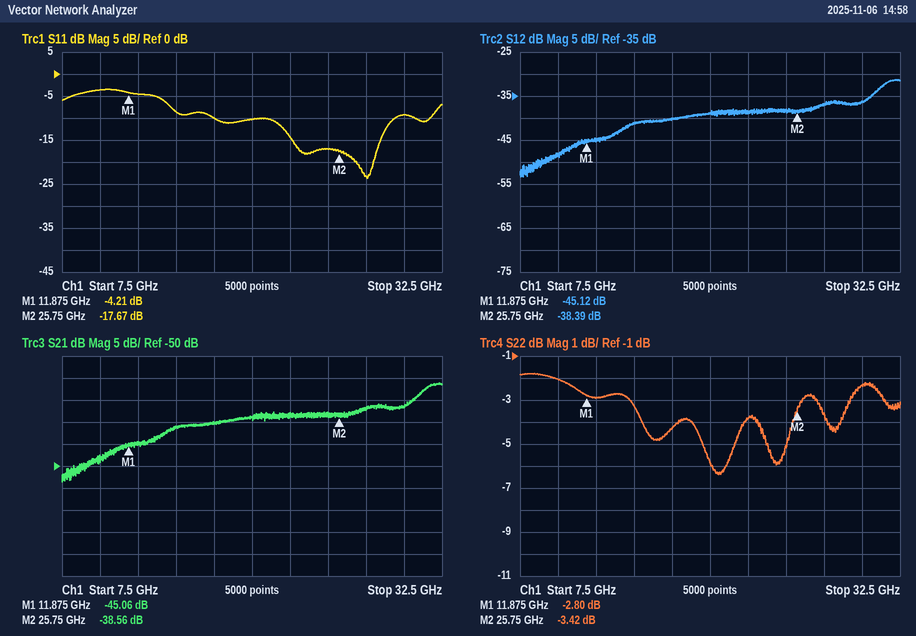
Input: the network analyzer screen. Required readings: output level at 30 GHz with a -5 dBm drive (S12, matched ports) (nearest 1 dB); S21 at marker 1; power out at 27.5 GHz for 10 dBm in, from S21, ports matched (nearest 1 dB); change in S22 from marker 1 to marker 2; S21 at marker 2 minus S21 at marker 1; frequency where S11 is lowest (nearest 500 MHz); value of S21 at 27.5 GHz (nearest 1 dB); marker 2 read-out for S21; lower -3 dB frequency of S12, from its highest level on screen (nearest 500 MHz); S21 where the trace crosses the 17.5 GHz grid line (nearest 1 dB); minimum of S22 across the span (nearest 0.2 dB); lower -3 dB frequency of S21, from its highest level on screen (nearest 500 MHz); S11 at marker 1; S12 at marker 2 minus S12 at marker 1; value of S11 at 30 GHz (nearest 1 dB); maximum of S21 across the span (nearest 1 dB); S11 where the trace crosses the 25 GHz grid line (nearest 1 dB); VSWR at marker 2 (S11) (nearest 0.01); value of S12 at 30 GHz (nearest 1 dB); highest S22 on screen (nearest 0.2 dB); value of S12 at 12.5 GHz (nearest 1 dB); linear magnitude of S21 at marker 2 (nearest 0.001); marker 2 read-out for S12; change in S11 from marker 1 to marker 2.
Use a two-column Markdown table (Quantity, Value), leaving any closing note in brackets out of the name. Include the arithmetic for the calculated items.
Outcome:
| Quantity | Value |
|---|---|
| output level at 30 GHz with a -5 dBm drive (S12, matched ports) | -5 dBm + (-36 dB) = -41 dBm |
| S21 at marker 1 | -45.06 dB |
| power out at 27.5 GHz for 10 dBm in, from S21, ports matched | 10 dBm + (-37 dB) = -27 dBm |
| change in S22 from marker 1 to marker 2 | -3.42 − (-2.8) = -0.62 dB |
| S21 at marker 2 minus S21 at marker 1 | -38.56 − (-45.06) = 6.50 dB |
| frequency where S11 is lowest | 27.5 GHz |
| value of S21 at 27.5 GHz | -37 dB |
| marker 2 read-out for S21 | -38.56 dB |
| lower -3 dB frequency of S12, from its highest level on screen | 31.0 GHz |
| S21 where the trace crosses the 17.5 GHz grid line | -40 dB |
| minimum of S22 across the span | -6.4 dB |
| lower -3 dB frequency of S21, from its highest level on screen | 31.0 GHz |
| S11 at marker 1 | -4.21 dB |
| S12 at marker 2 minus S12 at marker 1 | -38.39 − (-45.12) = 6.73 dB |
| value of S11 at 30 GHz | -9 dB |
| maximum of S21 across the span | -31 dB |
| S11 where the trace crosses the 25 GHz grid line | -17 dB |
| VSWR at marker 2 (S11) | (1 + 0.1308)/(1 − 0.1308) ≈ 1.30 |
| value of S12 at 30 GHz | -36 dB |
| highest S22 on screen | -1.8 dB |
| value of S12 at 12.5 GHz | -45 dB |
| linear magnitude of S21 at marker 2 | 10^(-38.56/20) ≈ 0.012 |
| marker 2 read-out for S12 | -38.39 dB |
| change in S11 from marker 1 to marker 2 | -17.67 − (-4.21) = -13.46 dB |
